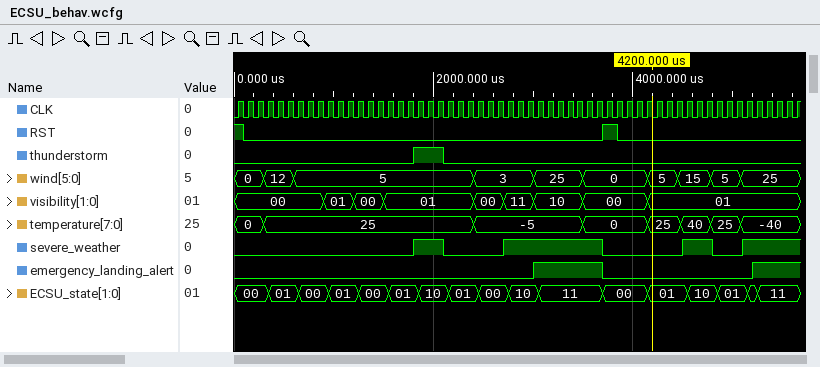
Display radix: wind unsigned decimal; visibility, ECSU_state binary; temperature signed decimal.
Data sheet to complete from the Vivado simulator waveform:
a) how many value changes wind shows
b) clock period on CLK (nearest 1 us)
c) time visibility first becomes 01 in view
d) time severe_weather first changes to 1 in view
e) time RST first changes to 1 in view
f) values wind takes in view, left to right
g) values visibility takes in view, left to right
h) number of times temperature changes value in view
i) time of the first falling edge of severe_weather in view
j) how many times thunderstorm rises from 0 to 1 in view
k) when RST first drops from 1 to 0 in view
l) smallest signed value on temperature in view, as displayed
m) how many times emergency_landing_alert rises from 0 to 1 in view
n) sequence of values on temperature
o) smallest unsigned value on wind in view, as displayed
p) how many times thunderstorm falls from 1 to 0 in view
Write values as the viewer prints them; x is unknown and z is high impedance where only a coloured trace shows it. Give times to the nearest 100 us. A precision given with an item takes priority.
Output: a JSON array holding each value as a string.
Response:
["9", "100 us", "900 us", "1800 us", "3700 us", "0, 12, 5, 3, 25, 0, 5, 15, 5, 25", "00, 01, 00, 01, 00, 11, 10, 00, 01", "7", "2100 us", "1", "100 us", "-40", "2", "0, 25, -5, 0, 25, 40, 25, -40", "0", "1"]
